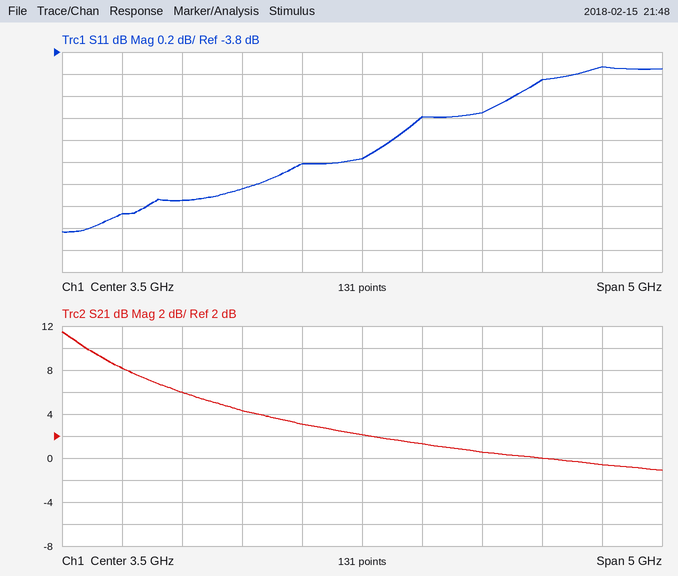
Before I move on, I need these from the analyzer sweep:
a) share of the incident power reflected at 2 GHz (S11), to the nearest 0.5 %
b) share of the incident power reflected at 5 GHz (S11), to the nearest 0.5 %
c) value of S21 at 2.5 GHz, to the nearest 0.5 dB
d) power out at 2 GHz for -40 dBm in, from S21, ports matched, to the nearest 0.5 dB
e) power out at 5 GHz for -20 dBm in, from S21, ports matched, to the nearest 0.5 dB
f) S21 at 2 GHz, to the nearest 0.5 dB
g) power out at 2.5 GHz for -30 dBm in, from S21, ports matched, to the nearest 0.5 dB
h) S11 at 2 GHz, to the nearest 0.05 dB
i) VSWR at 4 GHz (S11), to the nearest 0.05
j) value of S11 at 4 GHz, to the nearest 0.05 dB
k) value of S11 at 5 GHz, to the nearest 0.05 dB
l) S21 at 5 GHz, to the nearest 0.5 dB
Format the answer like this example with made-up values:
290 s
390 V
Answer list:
30.5 %
39.5 %
4.5 dB
-34.0 dBm
-20.0 dBm
6.0 dB
-25.5 dBm
-5.15 dB
4.05
-4.40 dB
-4.05 dB
0.0 dB
